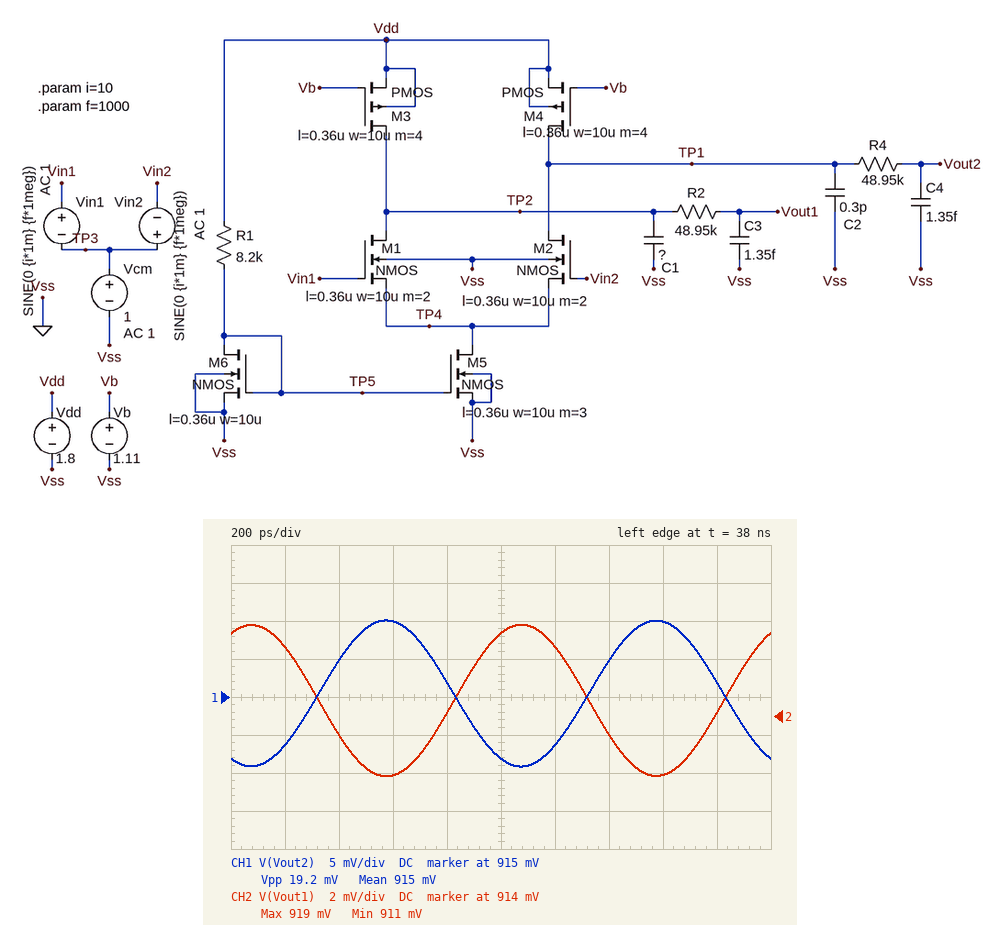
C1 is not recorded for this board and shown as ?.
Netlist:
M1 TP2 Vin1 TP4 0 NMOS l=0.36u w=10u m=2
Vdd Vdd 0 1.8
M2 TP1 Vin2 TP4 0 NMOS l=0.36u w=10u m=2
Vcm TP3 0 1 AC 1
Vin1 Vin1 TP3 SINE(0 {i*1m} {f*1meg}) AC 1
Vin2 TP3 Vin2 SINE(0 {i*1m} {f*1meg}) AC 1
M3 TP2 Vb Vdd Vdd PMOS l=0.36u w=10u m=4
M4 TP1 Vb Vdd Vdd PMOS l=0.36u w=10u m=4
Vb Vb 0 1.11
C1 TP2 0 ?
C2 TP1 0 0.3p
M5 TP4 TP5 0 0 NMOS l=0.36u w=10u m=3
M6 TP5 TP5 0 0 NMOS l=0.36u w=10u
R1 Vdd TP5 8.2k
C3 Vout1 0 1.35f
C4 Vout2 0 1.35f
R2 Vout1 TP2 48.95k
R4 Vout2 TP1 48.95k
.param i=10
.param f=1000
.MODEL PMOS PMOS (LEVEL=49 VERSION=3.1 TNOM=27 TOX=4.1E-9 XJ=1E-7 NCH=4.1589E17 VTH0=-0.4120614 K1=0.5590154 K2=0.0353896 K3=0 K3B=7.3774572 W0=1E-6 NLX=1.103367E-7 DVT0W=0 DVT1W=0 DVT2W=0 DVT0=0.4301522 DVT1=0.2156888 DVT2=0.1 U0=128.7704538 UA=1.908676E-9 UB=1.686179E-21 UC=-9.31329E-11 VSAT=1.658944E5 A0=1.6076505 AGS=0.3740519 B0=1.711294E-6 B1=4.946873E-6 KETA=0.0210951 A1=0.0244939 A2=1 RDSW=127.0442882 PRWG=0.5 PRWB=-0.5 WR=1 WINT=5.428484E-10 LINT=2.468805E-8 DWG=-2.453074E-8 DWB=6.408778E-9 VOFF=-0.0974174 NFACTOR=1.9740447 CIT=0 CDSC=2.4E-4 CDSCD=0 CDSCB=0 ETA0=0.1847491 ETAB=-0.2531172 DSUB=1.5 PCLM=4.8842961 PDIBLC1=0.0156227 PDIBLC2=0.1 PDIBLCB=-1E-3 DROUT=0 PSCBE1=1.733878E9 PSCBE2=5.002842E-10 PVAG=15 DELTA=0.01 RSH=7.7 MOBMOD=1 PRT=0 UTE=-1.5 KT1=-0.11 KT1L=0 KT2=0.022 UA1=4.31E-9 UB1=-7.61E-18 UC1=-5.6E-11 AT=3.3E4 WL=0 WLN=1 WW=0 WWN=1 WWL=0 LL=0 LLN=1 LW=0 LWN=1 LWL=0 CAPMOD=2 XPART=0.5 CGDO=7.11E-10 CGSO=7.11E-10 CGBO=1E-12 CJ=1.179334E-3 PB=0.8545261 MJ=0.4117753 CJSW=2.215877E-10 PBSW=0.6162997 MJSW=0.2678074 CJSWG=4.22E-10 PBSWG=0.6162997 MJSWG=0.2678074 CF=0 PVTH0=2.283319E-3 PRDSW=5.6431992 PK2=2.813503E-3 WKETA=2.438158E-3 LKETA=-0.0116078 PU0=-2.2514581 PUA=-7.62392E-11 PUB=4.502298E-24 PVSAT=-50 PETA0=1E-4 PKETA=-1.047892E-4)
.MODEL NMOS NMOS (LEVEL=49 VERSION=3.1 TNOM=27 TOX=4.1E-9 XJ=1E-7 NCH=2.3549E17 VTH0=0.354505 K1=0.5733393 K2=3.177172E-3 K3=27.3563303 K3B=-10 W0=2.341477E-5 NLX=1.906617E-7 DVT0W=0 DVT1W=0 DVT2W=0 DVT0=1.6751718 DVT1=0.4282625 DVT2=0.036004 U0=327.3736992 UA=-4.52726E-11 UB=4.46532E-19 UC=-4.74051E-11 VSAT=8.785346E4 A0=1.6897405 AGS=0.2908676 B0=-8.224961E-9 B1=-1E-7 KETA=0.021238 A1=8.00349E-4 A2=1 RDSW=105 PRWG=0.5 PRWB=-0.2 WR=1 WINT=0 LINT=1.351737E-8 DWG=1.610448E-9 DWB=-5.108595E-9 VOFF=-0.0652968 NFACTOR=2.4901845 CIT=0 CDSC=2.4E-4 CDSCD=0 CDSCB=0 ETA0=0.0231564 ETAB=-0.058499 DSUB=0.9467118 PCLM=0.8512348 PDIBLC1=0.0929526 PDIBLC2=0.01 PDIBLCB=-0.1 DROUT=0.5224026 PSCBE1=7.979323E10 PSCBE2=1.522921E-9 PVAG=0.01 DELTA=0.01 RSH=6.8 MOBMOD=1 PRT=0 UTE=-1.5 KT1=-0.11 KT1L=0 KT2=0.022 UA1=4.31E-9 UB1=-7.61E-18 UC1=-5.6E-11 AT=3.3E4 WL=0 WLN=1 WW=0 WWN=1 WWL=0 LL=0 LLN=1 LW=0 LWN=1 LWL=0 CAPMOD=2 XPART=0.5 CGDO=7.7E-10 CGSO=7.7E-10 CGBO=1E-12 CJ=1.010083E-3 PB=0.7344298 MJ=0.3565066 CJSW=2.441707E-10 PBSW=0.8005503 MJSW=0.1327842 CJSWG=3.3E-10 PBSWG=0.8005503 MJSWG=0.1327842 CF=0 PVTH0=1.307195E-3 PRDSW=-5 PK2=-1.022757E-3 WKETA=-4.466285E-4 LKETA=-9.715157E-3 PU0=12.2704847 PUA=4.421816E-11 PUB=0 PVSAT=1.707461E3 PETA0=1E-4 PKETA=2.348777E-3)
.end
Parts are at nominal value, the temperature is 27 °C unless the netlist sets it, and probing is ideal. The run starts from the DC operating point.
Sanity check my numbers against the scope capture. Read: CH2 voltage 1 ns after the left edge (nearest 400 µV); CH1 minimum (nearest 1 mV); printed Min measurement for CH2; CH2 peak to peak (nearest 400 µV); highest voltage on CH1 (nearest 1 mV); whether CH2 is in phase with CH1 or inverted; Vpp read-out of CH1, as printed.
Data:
918.4 mV
906 mV
911 mV
8.0 mV
925 mV
inverted
19.2 mV
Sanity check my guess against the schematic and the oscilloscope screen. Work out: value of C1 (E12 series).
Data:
820 fF
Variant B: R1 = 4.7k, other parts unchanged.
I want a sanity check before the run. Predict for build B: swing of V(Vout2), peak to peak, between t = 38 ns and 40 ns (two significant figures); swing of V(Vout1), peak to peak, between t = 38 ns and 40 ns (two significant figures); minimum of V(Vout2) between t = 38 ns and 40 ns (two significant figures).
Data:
2.3 mV
1.1 mV
130 mV
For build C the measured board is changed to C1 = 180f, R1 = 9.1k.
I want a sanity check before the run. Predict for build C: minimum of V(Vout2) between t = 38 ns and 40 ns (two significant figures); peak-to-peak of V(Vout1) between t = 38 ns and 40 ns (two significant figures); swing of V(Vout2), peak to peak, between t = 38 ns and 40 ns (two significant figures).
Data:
1.6 V
29 mV
18 mV
